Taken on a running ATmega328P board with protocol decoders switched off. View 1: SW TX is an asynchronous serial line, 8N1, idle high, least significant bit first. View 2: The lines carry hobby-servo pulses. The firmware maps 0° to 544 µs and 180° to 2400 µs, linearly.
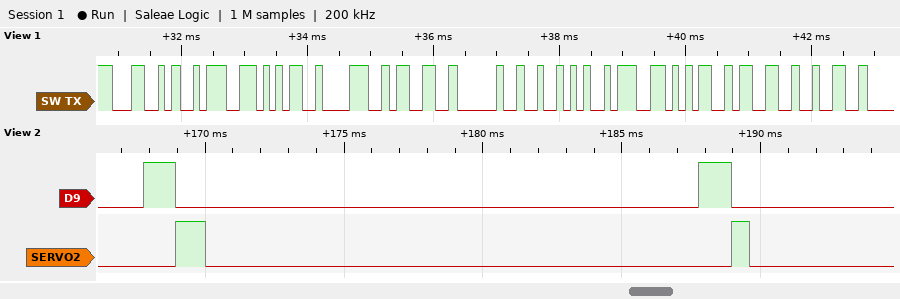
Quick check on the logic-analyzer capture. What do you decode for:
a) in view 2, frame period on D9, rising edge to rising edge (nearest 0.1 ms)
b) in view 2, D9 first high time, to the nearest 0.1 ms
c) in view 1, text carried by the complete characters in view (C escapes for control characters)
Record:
20.0 ms
1.2 ms
"L:583 R:532"
